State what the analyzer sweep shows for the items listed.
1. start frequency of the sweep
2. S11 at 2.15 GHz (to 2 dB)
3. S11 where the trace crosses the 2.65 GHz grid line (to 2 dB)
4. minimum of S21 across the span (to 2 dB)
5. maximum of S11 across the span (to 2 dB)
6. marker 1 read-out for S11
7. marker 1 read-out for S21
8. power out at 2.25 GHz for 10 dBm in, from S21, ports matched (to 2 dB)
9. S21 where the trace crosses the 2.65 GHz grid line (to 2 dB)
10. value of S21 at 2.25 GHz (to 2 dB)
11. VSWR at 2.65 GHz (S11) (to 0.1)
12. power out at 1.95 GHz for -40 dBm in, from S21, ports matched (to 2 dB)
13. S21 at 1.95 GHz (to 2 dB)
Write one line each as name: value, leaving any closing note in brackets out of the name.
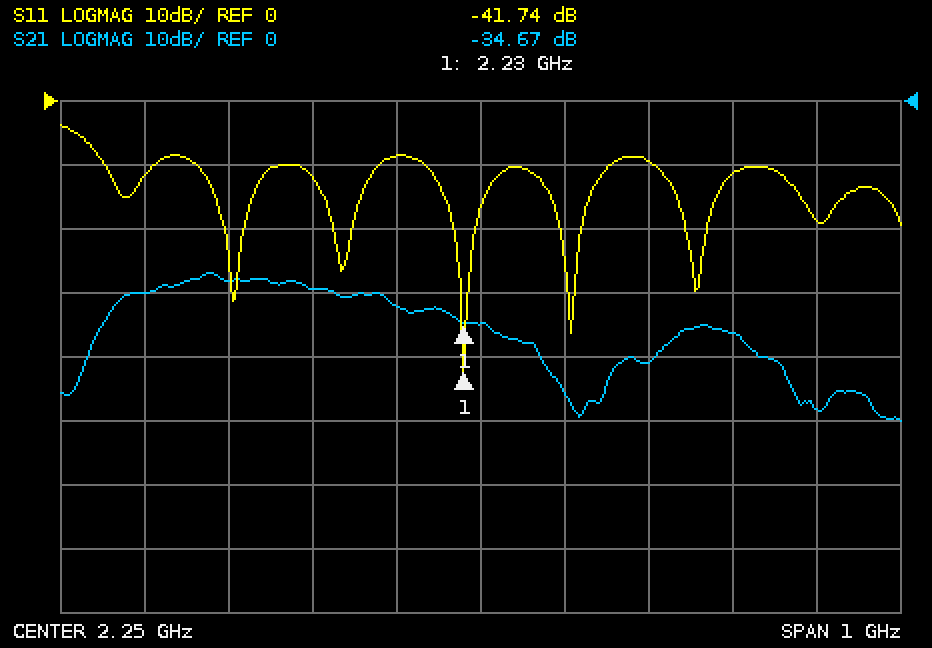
start frequency of the sweep: 1.75 GHz
S11 at 2.15 GHz: -8 dB
S11 where the trace crosses the 2.65 GHz grid line: -18 dB
minimum of S21 across the span: -50 dB
maximum of S11 across the span: -4 dB
marker 1 read-out for S11: -41.74 dB
marker 1 read-out for S21: -34.67 dB
power out at 2.25 GHz for 10 dBm in, from S21, ports matched: -24 dBm
S21 where the trace crosses the 2.65 GHz grid line: -48 dB
value of S21 at 2.25 GHz: -34 dB
VSWR at 2.65 GHz (S11): 1.3
power out at 1.95 GHz for -40 dBm in, from S21, ports matched: -68 dBm
S21 at 1.95 GHz: -28 dB
